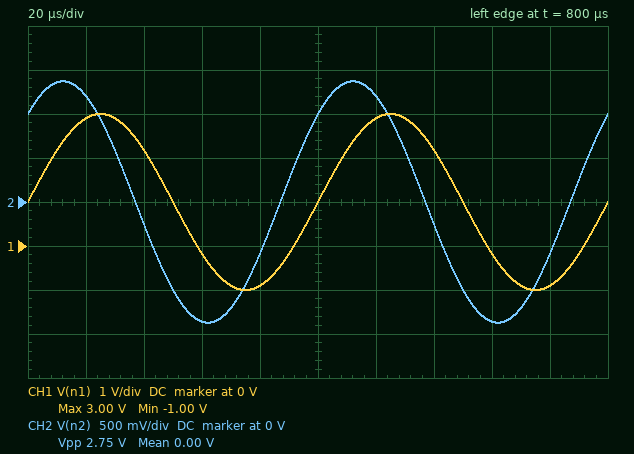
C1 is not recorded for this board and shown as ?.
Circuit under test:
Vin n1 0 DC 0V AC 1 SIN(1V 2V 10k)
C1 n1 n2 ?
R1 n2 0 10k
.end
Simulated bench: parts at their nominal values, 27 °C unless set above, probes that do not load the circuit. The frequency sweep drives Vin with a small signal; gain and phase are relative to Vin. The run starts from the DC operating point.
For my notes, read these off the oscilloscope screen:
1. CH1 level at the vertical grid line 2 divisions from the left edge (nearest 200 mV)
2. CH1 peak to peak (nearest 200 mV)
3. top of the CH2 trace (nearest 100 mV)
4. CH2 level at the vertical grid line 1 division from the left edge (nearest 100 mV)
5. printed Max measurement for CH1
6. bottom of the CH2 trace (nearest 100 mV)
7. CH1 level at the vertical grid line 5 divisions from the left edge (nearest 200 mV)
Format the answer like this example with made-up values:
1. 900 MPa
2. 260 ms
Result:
1. 2.2 V
2. 4.0 V
3. 1.4 V
4. 1.2 V
5. 3.00 V
6. -1.4 V
7. 1.0 V
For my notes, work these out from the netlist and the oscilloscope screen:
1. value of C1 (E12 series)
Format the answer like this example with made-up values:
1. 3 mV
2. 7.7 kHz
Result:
1. 1.5 nF
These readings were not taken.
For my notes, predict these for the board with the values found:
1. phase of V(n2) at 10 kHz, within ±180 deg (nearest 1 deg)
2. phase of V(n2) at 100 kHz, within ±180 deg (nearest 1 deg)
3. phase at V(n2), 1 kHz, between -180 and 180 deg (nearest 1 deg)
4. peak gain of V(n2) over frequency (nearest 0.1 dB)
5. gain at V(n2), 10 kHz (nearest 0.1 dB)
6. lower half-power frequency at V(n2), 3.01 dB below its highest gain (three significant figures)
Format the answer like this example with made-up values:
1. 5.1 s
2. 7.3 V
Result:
1. 47 deg
2. 6 deg
3. 85 deg
4. 0 dB
5. -3.3 dB
6. 10.6 kHz
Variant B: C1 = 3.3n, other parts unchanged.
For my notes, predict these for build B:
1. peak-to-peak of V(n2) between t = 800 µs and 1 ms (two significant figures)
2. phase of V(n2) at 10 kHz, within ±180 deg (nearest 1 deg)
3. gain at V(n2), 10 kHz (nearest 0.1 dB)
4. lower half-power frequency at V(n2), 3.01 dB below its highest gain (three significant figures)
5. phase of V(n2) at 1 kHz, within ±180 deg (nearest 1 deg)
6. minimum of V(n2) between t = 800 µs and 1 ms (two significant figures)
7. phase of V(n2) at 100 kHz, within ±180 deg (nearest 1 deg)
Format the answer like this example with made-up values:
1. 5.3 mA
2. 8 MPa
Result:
1. 3.6 V
2. 26 deg
3. -0.9 dB
4. 4.82 kHz
5. 78 deg
6. -1.8 V
7. 3 deg
